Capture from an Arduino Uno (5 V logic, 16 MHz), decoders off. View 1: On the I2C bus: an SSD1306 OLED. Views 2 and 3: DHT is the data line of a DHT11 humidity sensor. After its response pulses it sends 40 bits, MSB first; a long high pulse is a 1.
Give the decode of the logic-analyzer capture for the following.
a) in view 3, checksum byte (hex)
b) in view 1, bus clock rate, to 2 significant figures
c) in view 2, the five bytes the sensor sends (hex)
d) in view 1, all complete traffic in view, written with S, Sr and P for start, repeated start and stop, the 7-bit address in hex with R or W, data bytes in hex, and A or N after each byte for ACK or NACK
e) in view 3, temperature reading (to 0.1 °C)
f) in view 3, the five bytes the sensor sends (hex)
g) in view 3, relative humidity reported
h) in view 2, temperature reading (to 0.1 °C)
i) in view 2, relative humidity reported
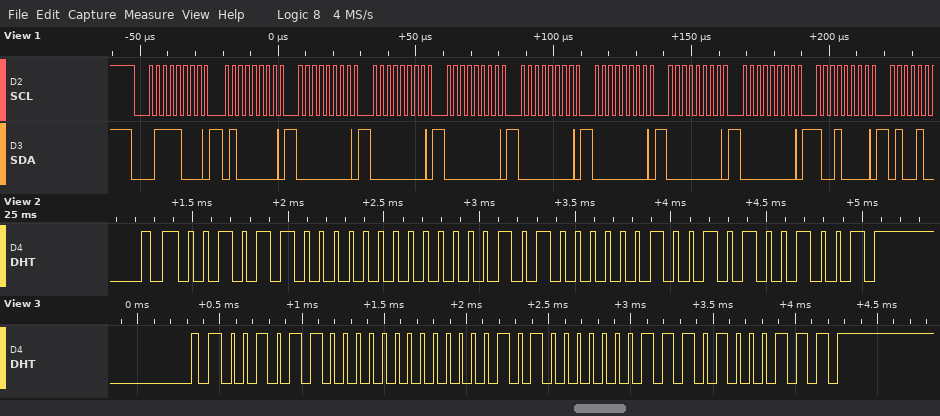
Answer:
0x47
400 kHz
2C 00 14 09 49
S 3CW A 40 A 00 A 00 A 00 A 00 A 00 A 00 A 00 A 90 A
20.7 °C
2C 00 14 07 47
44 %
20.9 °C
44 %
